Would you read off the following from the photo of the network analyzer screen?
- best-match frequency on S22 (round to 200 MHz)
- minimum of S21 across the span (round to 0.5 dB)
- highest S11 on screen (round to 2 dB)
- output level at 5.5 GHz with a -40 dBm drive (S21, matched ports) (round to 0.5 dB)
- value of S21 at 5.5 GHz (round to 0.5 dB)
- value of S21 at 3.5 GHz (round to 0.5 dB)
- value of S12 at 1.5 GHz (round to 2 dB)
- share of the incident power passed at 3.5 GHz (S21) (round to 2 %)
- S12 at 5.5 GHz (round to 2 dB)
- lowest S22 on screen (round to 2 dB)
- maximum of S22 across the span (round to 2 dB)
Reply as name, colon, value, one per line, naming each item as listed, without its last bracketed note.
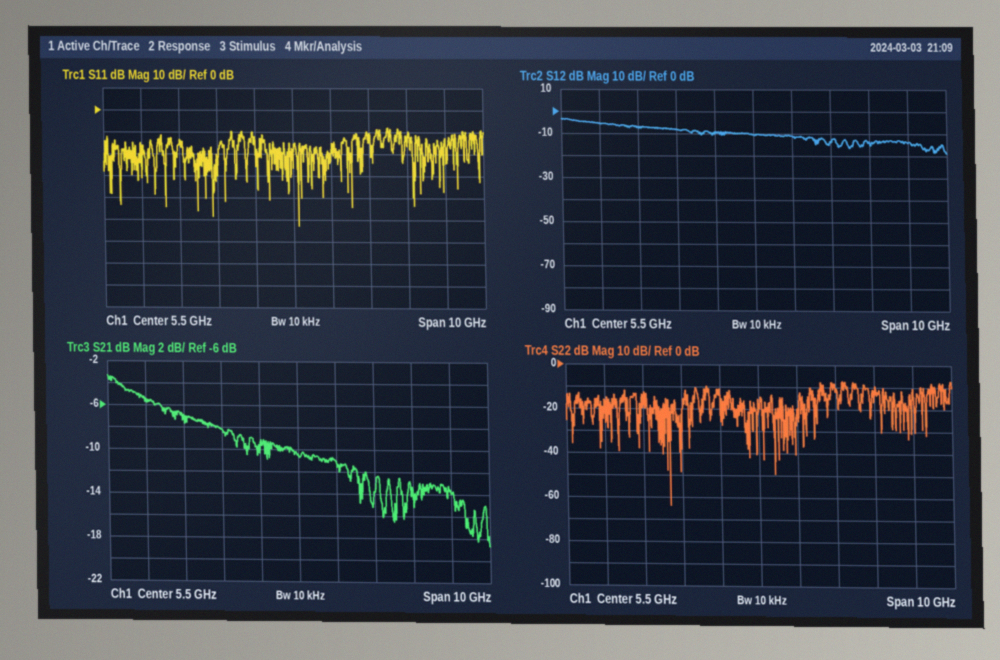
best-match frequency on S22: 3.2 GHz
minimum of S21 across the span: -18.5 dB
highest S11 on screen: -8 dB
output level at 5.5 GHz with a -40 dBm drive (S21, matched ports): -50.5 dBm
value of S21 at 5.5 GHz: -10.5 dB
value of S21 at 3.5 GHz: -8.0 dB
value of S12 at 1.5 GHz: -6 dB
share of the incident power passed at 3.5 GHz (S21): 16 %
S12 at 5.5 GHz: -10 dB
lowest S22 on screen: -64 dB
maximum of S22 across the span: -8 dB
